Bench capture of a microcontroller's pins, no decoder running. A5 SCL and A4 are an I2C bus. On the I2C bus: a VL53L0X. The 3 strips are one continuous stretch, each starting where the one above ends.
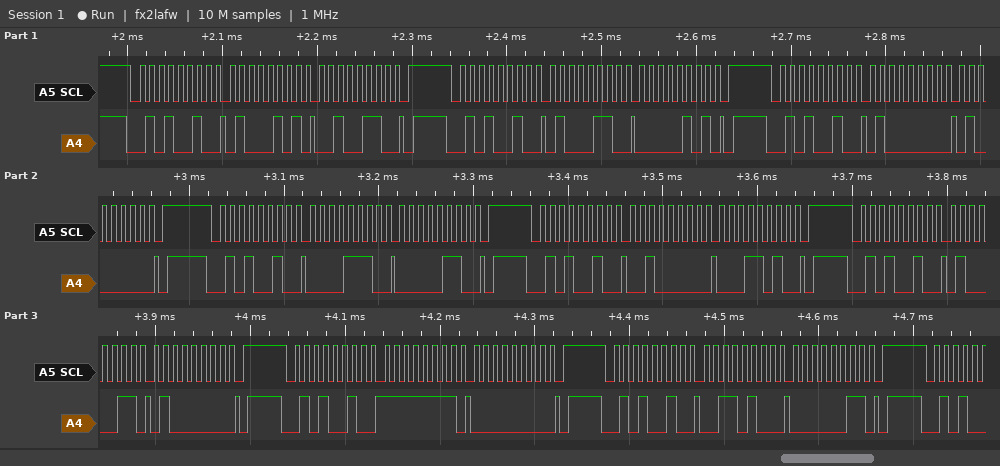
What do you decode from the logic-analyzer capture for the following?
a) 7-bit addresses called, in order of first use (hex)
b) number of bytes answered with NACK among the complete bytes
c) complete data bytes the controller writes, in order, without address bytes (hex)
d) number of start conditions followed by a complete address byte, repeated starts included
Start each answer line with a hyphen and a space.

- 0x29
- 0
- 45 26 46 05 40 40 0E 06 20 1A 43 40 FF 00 34 03
- 8
